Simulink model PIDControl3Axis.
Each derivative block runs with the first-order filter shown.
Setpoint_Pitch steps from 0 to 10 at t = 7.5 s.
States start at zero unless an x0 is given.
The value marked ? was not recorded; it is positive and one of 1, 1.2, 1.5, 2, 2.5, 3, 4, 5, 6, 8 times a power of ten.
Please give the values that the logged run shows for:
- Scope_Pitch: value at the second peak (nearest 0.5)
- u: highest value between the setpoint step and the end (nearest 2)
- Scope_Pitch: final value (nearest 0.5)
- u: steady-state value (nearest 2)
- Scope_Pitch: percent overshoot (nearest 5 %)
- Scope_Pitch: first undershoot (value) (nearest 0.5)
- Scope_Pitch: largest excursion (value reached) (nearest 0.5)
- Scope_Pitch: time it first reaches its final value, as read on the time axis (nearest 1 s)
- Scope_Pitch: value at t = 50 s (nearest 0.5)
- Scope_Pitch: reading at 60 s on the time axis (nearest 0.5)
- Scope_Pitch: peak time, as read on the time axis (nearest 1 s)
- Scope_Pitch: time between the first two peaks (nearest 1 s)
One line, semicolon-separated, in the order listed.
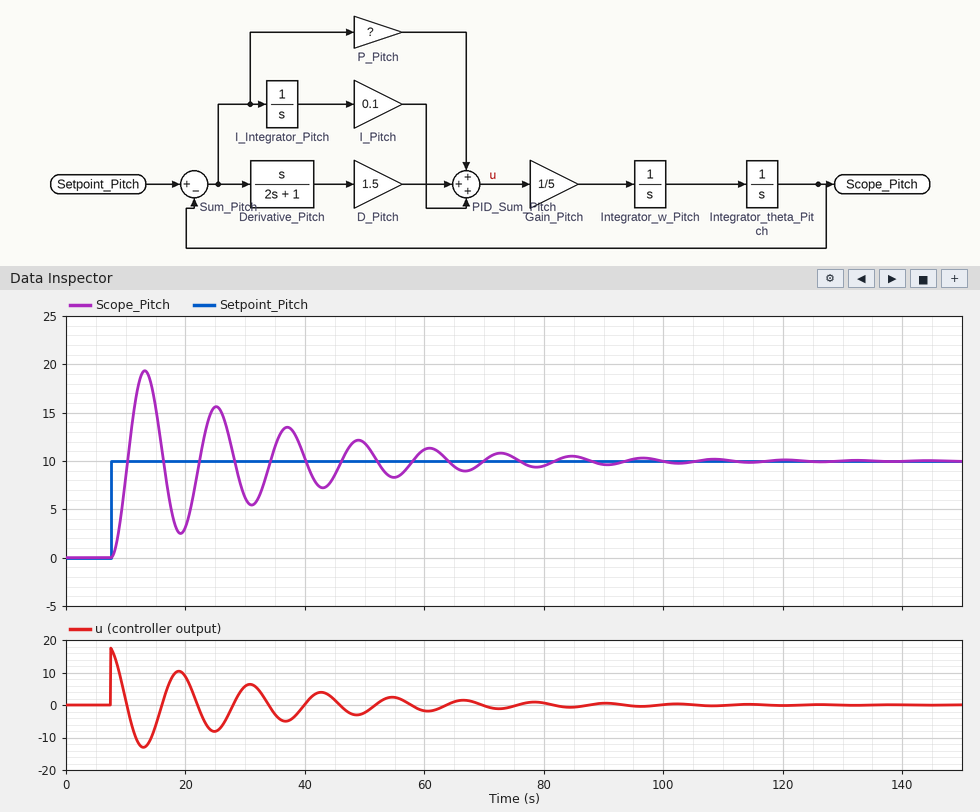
15.5; 18; 10.0; 0; 95 %; 2.5; 19.5; 10 s; 12.0; 11.0; 13 s; 12 s
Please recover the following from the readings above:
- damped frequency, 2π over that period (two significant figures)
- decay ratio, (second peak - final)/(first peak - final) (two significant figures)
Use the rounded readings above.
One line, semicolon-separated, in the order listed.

0.52 rad/s; 0.58
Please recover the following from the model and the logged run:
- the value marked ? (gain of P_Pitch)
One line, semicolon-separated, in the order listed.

1
